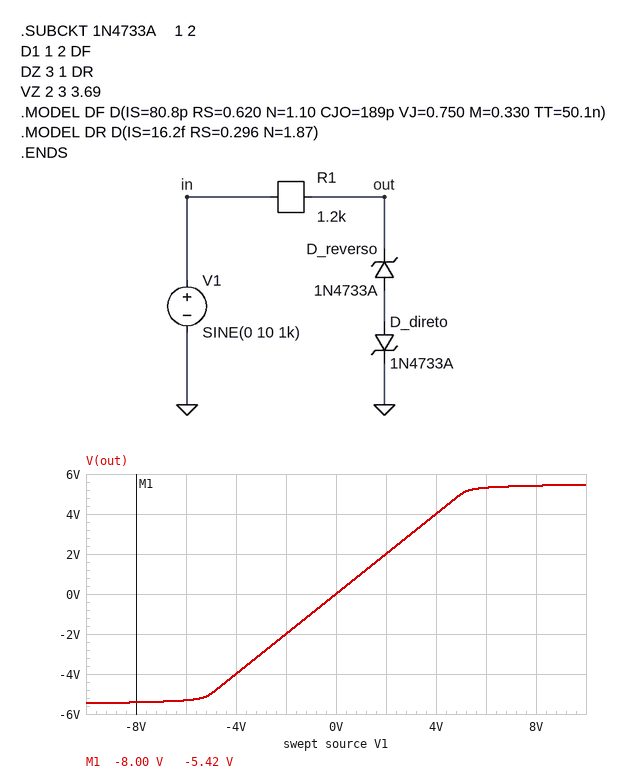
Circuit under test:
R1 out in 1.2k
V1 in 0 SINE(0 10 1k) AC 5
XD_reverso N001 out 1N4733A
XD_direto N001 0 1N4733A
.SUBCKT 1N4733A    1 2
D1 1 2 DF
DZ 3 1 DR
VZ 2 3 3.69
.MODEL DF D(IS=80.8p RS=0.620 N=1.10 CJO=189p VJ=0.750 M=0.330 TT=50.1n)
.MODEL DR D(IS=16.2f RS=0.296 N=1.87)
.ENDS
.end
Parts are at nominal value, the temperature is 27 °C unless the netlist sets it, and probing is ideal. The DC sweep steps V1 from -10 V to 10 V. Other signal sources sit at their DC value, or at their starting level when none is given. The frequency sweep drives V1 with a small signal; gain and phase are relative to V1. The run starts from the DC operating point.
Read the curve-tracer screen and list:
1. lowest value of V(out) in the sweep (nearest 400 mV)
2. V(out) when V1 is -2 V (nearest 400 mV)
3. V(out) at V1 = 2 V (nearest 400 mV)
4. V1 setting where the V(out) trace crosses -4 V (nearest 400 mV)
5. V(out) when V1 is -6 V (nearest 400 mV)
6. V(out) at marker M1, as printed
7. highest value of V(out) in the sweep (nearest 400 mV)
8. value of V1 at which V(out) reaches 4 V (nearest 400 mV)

-5.6 V
-2.0 V
2.0 V
-4.0 V
-5.2 V
-5.42 V
5.6 V
4.0 V
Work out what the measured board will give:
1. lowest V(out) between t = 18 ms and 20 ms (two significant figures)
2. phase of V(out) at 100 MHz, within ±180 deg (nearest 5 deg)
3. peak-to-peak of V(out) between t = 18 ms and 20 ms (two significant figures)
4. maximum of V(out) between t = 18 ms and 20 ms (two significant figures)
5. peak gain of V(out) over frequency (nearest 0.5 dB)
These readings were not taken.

-5.5 V
-85 deg
11 V
5.5 V
0 dB
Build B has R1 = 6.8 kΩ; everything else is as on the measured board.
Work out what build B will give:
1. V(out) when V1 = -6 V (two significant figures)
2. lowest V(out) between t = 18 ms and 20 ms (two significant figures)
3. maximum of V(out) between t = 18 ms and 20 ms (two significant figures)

-5.2 V
-5.3 V
5.3 V
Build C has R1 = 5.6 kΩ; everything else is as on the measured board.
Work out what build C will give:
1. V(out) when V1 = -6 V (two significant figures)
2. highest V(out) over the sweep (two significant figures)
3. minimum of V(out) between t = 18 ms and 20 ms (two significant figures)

-5.2 V
5.3 V
-5.3 V
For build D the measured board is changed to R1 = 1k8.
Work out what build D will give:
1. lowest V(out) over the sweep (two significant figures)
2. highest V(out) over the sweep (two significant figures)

-5.4 V
5.4 V
